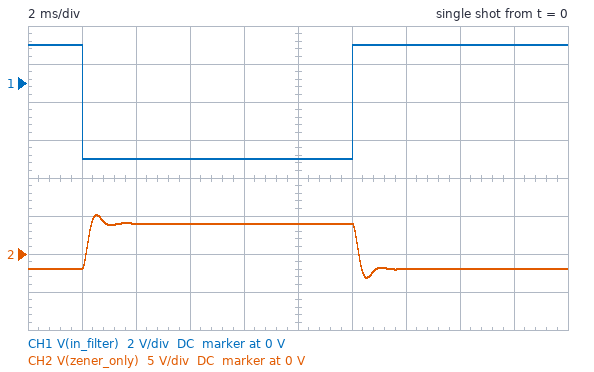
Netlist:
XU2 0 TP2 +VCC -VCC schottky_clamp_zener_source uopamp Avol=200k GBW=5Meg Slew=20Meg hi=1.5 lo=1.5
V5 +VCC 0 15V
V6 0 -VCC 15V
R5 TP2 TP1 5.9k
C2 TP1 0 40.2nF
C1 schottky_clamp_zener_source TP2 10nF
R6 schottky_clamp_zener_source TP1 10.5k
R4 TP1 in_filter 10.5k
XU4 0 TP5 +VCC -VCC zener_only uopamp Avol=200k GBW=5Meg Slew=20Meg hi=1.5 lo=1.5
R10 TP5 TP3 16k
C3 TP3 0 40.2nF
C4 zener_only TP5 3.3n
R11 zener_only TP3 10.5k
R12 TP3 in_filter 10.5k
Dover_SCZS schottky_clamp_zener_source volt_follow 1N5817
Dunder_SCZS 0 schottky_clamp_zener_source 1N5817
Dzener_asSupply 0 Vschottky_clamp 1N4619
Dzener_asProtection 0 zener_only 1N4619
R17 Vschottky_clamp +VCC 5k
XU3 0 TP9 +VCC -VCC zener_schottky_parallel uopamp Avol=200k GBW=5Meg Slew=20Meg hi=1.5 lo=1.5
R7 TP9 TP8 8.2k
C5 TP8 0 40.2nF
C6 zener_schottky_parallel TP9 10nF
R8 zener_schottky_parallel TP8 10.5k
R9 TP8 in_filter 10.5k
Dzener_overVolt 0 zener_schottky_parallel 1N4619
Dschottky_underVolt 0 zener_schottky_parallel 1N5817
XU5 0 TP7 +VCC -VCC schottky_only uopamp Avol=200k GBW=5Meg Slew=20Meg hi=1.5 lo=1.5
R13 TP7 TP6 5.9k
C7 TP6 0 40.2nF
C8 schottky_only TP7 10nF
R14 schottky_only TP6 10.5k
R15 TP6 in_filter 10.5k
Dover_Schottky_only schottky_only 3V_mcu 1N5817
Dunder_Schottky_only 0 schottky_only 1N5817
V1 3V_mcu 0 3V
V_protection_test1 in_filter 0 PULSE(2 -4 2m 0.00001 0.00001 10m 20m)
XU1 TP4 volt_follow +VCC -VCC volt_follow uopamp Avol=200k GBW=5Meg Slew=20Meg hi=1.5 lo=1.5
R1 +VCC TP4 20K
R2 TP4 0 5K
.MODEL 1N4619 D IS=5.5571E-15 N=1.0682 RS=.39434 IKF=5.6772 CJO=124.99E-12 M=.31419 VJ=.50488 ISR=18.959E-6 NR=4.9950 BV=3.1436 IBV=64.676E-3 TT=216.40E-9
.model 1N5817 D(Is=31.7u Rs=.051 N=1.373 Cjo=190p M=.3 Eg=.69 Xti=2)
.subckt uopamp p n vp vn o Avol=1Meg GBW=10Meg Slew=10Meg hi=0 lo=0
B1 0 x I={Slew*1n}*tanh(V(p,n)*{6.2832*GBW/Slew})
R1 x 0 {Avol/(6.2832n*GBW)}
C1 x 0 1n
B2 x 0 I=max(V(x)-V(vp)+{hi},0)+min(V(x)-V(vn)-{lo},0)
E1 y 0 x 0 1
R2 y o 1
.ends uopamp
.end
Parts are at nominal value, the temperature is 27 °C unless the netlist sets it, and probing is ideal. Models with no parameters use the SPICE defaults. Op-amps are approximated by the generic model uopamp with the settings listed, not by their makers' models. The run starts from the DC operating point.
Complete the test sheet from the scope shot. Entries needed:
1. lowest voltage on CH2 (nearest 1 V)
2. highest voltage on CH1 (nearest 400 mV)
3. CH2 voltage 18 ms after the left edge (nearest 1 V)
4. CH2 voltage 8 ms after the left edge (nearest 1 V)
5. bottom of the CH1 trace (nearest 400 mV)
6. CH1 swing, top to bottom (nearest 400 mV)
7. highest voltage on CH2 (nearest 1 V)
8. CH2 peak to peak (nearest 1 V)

-3 V
2.0 V
-2 V
4 V
-4.0 V
6.0 V
5 V
8 V
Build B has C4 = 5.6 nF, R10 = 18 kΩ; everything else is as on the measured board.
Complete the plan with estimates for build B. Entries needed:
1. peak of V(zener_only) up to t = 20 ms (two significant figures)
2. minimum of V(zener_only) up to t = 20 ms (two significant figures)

4.5 V
-2.5 V
